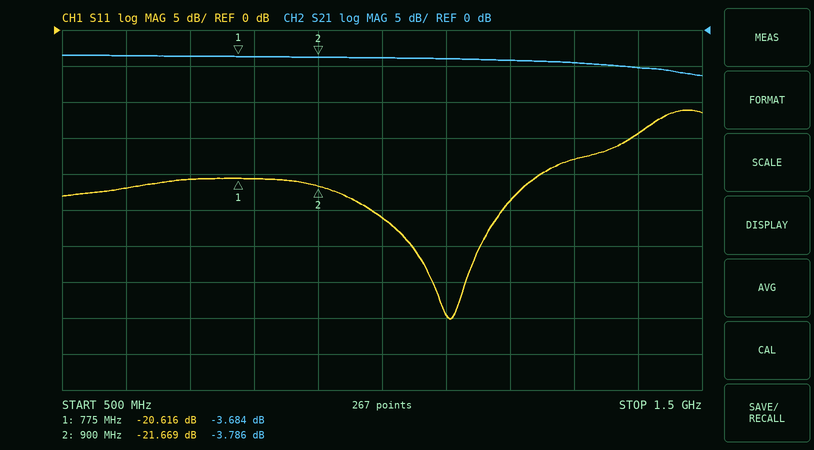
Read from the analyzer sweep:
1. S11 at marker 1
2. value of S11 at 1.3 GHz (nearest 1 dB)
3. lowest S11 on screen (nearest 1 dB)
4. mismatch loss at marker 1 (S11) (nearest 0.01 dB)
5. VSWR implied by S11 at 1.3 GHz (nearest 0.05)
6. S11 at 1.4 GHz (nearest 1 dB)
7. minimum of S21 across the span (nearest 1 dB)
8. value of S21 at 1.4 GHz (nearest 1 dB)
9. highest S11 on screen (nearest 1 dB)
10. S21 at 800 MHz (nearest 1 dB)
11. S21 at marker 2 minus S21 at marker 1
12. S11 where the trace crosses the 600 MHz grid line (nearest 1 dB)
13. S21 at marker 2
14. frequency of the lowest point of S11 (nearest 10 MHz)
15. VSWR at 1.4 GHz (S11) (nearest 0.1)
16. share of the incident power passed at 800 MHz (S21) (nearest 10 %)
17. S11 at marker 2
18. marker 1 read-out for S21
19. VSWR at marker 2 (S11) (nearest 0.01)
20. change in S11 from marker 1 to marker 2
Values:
-20.616 dB
-18 dB
-40 dB
0.04 dB
1.30
-14 dB
-6 dB
-5 dB
-11 dB
-4 dB
-0.102 dB
-22 dB
-3.786 dB
1.11 GHz
1.5
40 %
-21.669 dB
-3.684 dB
1.18
-1.053 dB
